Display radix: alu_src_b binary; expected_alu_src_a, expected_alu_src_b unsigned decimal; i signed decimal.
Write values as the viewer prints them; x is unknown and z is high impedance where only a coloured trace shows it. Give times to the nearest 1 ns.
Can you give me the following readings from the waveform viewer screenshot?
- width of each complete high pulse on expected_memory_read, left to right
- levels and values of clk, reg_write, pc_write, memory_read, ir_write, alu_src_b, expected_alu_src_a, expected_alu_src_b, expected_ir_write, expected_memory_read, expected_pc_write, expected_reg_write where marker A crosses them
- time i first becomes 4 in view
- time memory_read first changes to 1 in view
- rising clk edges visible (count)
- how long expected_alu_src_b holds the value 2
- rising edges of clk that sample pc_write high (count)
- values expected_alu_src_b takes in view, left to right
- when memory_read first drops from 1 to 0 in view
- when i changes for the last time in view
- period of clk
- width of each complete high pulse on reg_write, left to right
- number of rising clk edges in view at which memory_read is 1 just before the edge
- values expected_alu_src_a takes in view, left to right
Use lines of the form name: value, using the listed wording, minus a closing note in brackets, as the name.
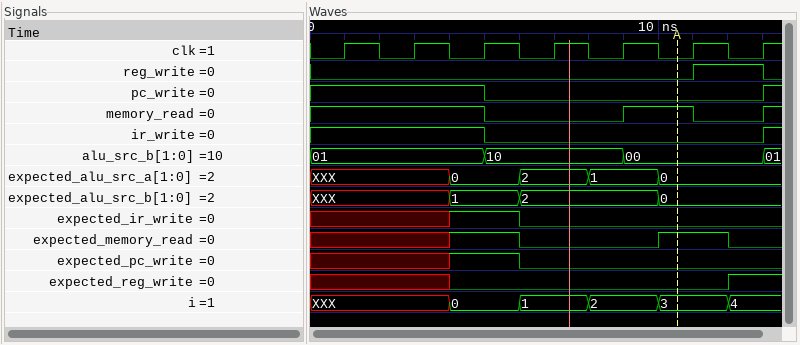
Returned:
width of each complete high pulse on expected_memory_read, left to right: 2 ns
levels and values of clk, reg_write, pc_write, memory_read, ir_write, alu_src_b, expected_alu_src_a, expected_alu_src_b, expected_ir_write, expected_memory_read, expected_pc_write, expected_reg_write where marker A crosses them: clk=0, reg_write=0, pc_write=0, memory_read=1, ir_write=0, alu_src_b=00, expected_alu_src_a=0, expected_alu_src_b=0, expected_ir_write=0, expected_memory_read=1, expected_pc_write=0, expected_reg_write=0
time i first becomes 4 in view: 12 ns
time memory_read first changes to 1 in view: 9 ns
rising clk edges visible: 7
how long expected_alu_src_b holds the value 2: 4 ns
rising edges of clk that sample pc_write high: 3
values expected_alu_src_b takes in view, left to right: XXX, 1, 2, 0
when memory_read first drops from 1 to 0 in view: 5 ns
when i changes for the last time in view: 12 ns
period of clk: 2 ns
width of each complete high pulse on reg_write, left to right: 2 ns
number of rising clk edges in view at which memory_read is 1 just before the edge: 4
values expected_alu_src_a takes in view, left to right: XXX, 0, 2, 1, 0
